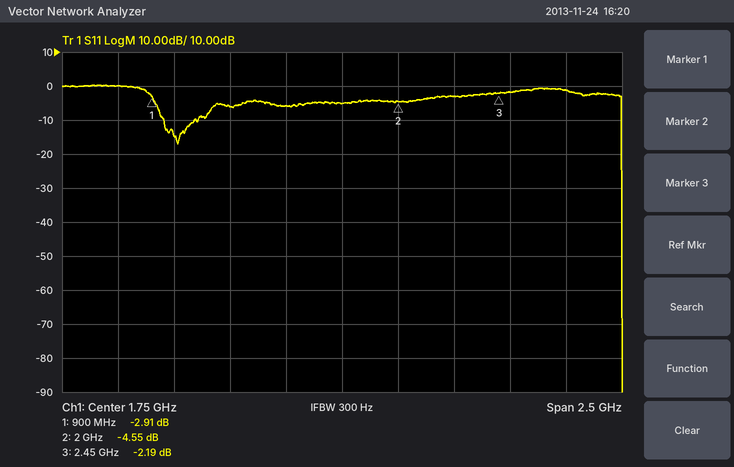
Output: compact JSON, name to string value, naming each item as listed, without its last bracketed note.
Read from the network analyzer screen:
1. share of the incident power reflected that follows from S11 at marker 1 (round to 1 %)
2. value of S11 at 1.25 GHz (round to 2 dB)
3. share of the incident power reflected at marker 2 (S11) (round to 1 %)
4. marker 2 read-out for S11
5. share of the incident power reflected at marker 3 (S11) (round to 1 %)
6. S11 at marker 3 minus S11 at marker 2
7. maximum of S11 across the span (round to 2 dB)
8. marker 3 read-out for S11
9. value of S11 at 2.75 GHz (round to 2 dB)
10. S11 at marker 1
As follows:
{"share of the incident power reflected that follows from S11 at marker 1": "51 %", "value of S11 at 1.25 GHz": "-6 dB", "share of the incident power reflected at marker 2 (S11)": "35 %", "marker 2 read-out for S11": "-4.55 dB", "share of the incident power reflected at marker 3 (S11)": "60 %", "S11 at marker 3 minus S11 at marker 2": "2.36 dB", "maximum of S11 across the span": "0 dB", "marker 3 read-out for S11": "-2.19 dB", "value of S11 at 2.75 GHz": "-2 dB", "S11 at marker 1": "-2.91 dB"}
